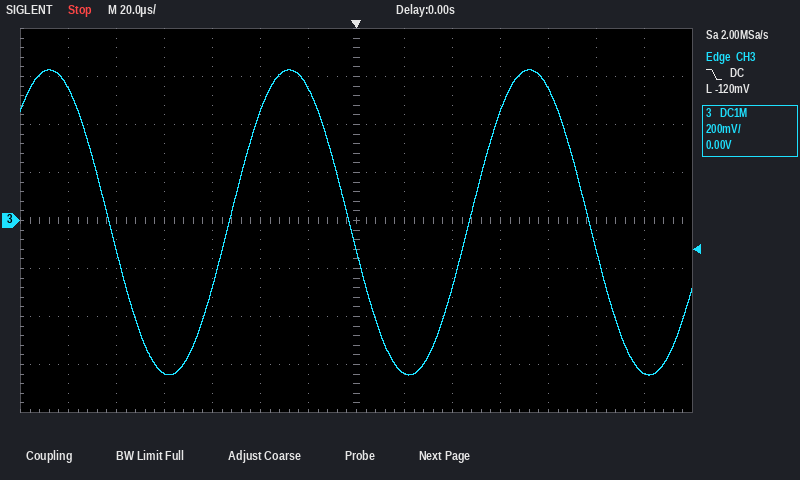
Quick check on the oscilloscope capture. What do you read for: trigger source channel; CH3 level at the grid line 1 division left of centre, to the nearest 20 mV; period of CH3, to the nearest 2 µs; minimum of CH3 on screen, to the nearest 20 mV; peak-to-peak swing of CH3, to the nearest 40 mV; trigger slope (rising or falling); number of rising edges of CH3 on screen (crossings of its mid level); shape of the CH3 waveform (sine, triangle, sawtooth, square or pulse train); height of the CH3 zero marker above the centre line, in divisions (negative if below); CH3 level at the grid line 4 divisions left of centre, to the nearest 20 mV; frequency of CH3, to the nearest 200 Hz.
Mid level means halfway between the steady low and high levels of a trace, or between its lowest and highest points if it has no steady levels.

CH3
560 mV
100 µs
-640 mV
1.28 V
falling
2
sine
0.0 div
-640 mV
10.0 kHz
